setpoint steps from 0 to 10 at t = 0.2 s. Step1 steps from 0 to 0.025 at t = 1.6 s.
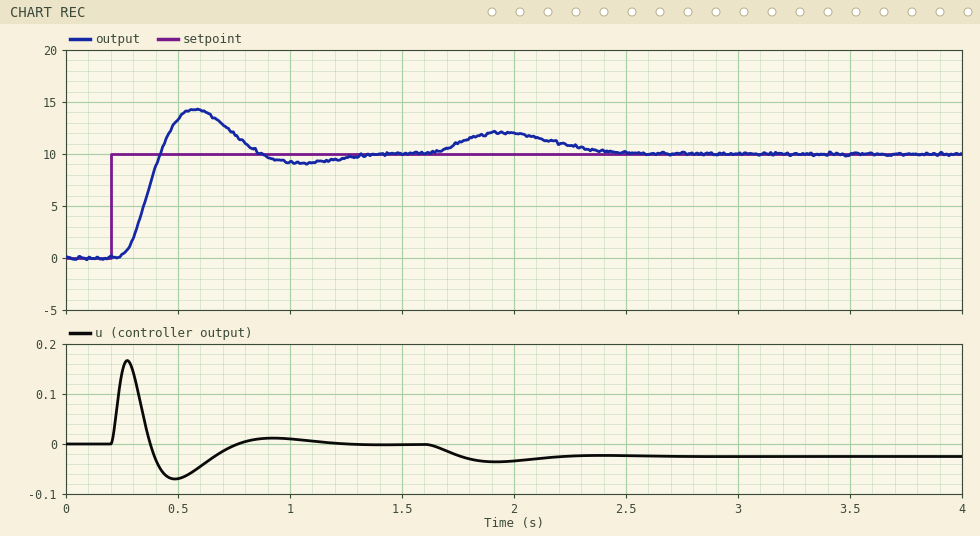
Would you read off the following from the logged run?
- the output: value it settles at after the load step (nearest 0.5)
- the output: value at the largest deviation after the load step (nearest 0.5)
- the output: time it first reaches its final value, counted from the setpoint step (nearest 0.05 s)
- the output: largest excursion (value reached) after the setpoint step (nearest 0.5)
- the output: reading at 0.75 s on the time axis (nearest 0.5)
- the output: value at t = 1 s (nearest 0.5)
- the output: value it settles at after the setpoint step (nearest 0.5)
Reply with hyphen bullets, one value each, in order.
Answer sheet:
- 10.0
- 12.0
- 0.20 s
- 14.5
- 12.0
- 9.0
- 10.0
